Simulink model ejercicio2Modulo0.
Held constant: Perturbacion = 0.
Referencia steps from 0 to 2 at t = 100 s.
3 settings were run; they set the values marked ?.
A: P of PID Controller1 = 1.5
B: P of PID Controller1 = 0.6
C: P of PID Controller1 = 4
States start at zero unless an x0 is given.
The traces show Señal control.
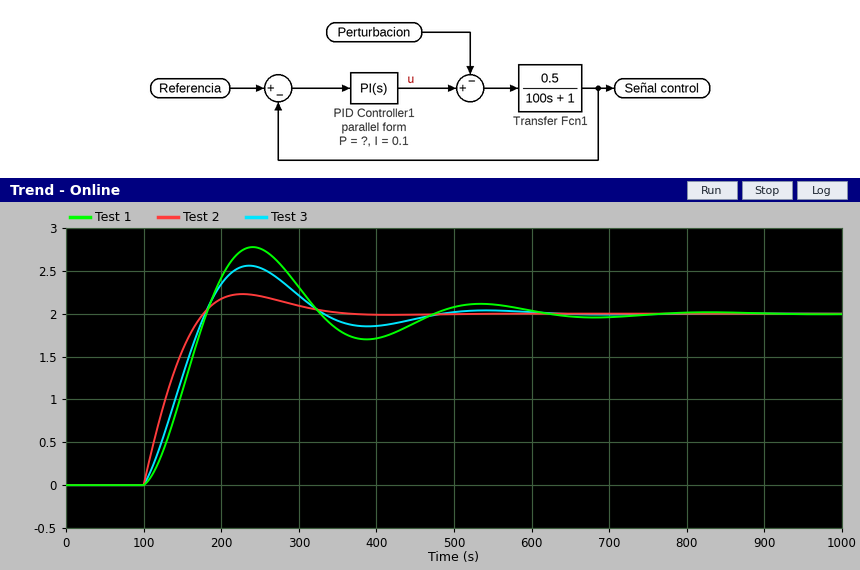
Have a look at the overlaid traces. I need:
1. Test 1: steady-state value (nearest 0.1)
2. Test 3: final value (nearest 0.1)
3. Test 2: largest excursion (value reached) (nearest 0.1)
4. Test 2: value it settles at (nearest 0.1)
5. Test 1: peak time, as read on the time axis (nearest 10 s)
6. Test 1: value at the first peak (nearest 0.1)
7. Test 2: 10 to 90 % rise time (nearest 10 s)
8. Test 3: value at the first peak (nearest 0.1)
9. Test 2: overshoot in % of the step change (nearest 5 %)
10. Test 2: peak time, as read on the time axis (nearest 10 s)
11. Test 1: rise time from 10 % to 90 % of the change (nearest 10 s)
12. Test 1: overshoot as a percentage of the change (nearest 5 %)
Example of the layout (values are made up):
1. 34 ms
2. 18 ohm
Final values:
1. 2.0
2. 2.0
3. 2.2
4. 2.0
5. 240 s
6. 2.8
7. 60 s
8. 2.6
9. 10 %
10. 230 s
11. 60 s
12. 40 %
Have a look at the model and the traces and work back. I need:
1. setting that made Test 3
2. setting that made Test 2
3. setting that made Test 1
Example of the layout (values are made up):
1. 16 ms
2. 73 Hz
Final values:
1. A
2. C
3. B
